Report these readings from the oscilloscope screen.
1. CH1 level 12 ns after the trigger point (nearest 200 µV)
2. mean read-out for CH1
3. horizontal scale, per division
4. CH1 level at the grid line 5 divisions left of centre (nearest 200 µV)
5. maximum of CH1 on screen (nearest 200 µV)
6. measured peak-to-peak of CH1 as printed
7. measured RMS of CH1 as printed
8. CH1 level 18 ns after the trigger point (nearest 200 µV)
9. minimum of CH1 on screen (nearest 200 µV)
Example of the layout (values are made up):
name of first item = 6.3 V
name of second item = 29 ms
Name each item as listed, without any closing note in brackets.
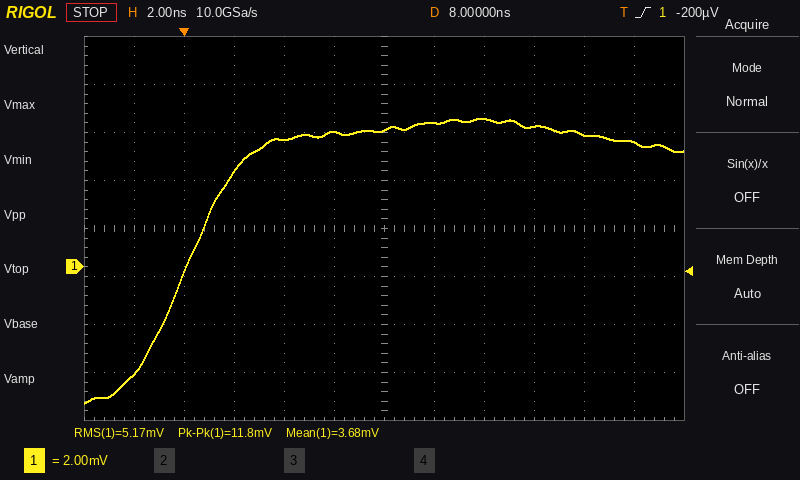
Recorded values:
CH1 level 12 ns after the trigger point = 6.2 mV
mean read-out for CH1 = 3.68 mV
horizontal scale, per division = 2 ns
CH1 level at the grid line 5 divisions left of centre = -4.4 mV
maximum of CH1 on screen = 6.2 mV
measured peak-to-peak of CH1 as printed = 11.8 mV
measured RMS of CH1 as printed = 5.17 mV
CH1 level 18 ns after the trigger point = 5.2 mV
minimum of CH1 on screen = -5.6 mV
